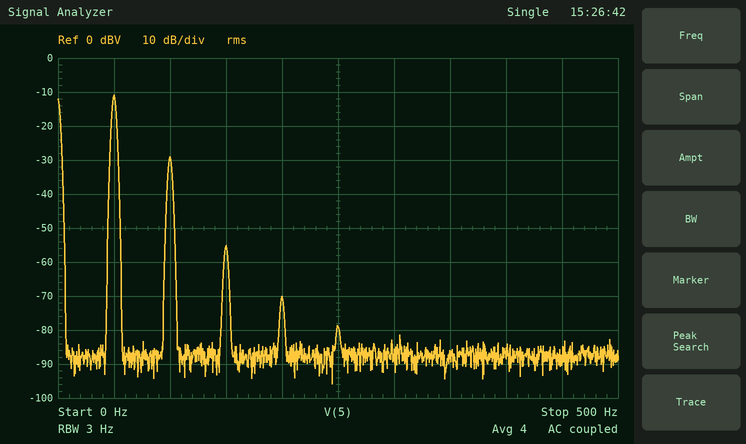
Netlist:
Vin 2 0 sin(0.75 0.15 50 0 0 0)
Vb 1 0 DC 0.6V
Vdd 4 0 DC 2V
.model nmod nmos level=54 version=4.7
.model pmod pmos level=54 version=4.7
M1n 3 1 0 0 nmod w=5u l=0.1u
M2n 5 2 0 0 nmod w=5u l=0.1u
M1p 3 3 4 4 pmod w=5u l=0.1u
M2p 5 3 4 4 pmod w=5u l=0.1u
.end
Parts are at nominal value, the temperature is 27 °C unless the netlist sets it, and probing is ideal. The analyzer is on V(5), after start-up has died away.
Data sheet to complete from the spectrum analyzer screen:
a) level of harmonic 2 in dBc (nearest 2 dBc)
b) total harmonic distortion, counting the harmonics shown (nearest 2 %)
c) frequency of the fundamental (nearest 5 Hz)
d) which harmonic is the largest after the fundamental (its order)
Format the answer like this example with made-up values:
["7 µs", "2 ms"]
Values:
["-18 dBc", "12 %", "50 Hz", "2"]
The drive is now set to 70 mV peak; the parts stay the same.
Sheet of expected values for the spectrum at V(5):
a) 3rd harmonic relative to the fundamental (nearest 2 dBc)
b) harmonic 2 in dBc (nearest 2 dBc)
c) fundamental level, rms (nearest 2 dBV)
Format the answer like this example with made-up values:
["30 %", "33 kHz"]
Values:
["-56 dBc", "-24 dBc", "-18 dBV"]
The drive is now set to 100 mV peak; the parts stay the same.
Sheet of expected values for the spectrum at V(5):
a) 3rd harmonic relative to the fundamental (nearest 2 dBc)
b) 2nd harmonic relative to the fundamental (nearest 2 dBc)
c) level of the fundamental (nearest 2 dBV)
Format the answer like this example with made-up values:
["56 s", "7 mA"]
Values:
["-50 dBc", "-22 dBc", "-14 dBV"]
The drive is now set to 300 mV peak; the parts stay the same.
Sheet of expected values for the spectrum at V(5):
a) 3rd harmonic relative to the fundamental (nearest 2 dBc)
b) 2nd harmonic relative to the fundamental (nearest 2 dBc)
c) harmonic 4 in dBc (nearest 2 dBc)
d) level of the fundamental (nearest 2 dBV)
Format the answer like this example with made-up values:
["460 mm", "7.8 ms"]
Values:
["-34 dBc", "-14 dBc", "-36 dBc", "-6 dBV"]
